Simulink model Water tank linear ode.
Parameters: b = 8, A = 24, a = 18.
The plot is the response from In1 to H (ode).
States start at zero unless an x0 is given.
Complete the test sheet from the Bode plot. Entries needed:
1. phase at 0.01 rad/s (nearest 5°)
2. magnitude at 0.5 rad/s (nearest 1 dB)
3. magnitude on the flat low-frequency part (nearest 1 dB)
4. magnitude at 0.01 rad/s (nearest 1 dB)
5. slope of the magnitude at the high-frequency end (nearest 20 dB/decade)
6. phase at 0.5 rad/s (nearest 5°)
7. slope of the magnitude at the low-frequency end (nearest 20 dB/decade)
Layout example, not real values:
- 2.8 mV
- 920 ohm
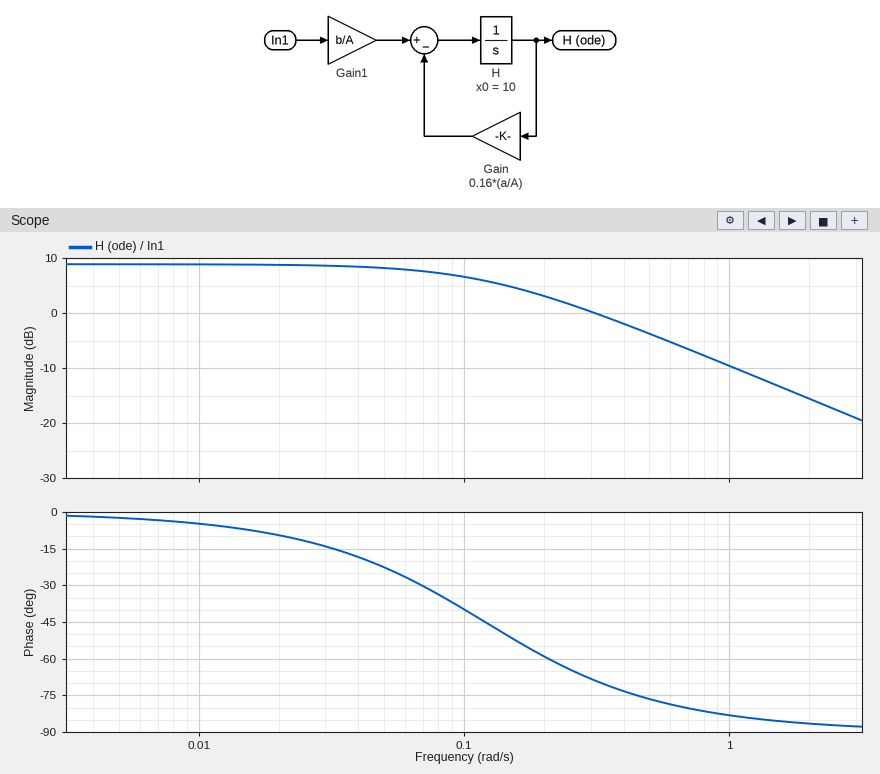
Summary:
- -5°
- -4 dB
- 9 dB
- 9 dB
- -20 dB/decade
- -75°
- 0 dB/decade
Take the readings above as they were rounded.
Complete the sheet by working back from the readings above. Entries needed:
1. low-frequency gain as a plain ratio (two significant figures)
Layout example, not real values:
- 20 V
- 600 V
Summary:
- 2.8
